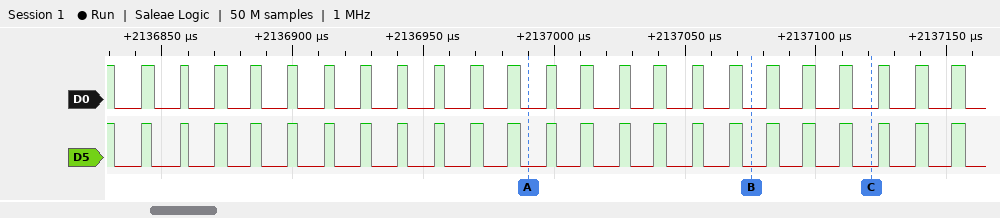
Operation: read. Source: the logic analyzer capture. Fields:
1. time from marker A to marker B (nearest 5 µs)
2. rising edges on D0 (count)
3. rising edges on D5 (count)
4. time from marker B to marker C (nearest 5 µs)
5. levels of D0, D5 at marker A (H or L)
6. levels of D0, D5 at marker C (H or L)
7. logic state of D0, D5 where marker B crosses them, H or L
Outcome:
85 µs
23
23
45 µs
D0=L, D5=L
D0=L, D5=L
D0=L, D5=L
